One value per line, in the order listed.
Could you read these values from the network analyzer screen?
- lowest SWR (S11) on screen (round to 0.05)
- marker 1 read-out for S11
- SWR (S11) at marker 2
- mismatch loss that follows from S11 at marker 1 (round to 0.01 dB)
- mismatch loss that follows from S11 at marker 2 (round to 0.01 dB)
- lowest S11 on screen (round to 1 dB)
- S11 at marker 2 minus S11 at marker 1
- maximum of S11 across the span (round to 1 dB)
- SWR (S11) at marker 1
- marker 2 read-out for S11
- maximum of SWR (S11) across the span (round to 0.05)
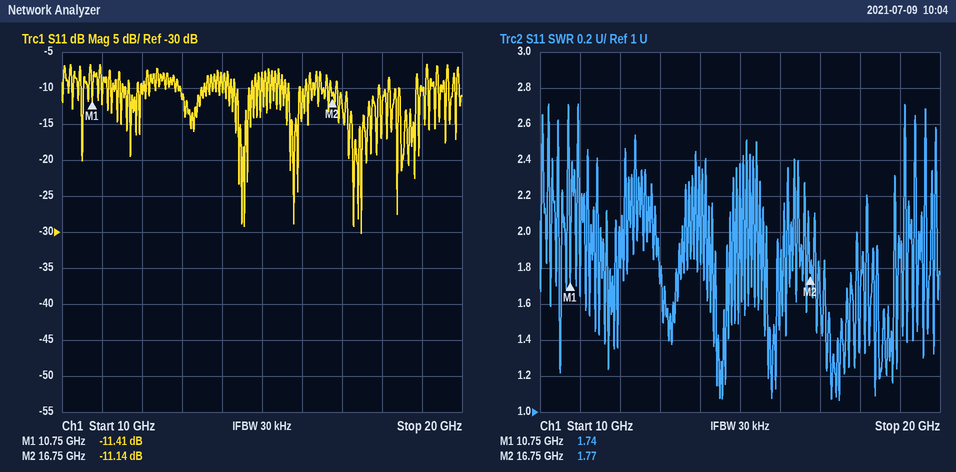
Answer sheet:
1.05
-11.41 dB
1.77
0.33 dB
0.35 dB
-30 dB
0.27 dB
-7 dB
1.74
-11.14 dB
2.70
